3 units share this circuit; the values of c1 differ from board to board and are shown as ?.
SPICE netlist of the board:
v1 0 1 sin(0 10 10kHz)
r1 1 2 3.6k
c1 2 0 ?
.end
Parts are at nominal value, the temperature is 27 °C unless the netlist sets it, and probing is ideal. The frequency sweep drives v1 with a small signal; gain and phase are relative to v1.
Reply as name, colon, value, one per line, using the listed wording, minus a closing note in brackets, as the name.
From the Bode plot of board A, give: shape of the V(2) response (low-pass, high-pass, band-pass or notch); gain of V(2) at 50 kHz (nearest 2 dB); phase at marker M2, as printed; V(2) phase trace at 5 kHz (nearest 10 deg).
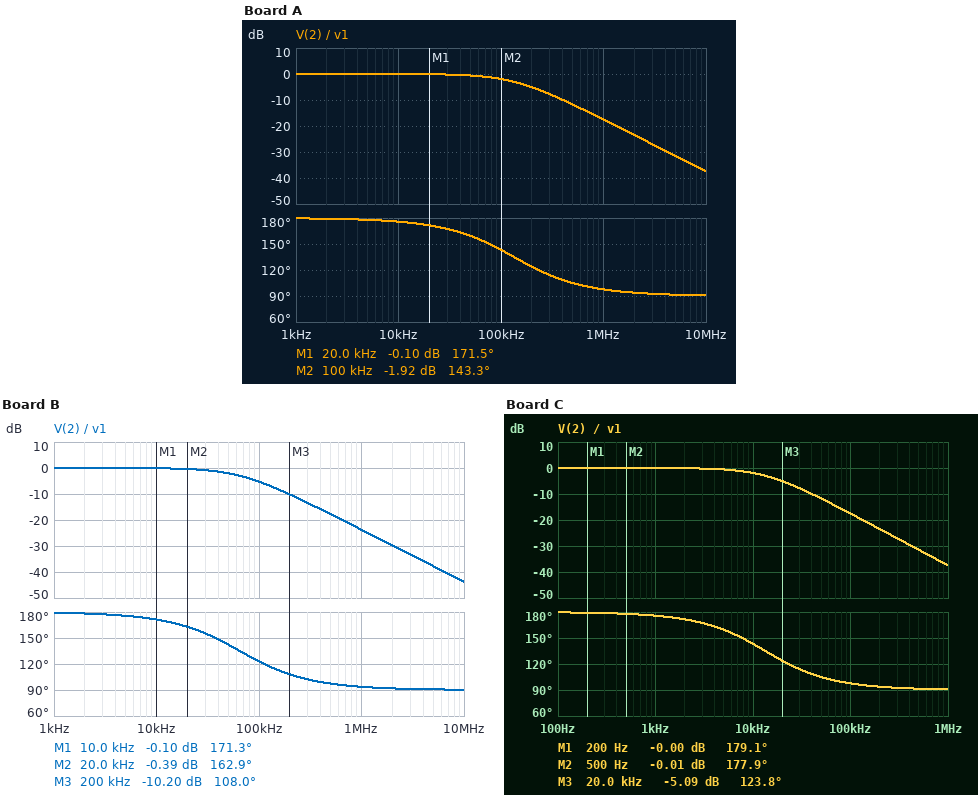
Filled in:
shape of the V(2) response: low-pass
gain of V(2) at 50 kHz: 0 dB
phase at marker M2, as printed: 143.3 deg
V(2) phase trace at 5 kHz: 180 deg
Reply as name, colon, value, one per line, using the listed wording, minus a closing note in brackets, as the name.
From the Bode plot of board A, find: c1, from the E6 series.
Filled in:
c1, from the E6 series: 330 pF
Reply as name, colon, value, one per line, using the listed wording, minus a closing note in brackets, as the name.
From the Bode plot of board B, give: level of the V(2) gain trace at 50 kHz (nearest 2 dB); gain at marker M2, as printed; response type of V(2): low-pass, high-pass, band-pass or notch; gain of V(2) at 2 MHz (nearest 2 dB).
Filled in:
level of the V(2) gain trace at 50 kHz: -2 dB
gain at marker M2, as printed: -0.39 dB
response type of V(2): low-pass, high-pass, band-pass or notch: low-pass
gain of V(2) at 2 MHz: -30 dB
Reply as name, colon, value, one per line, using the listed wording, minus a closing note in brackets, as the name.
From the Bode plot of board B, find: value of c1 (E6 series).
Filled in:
value of c1: 680 pF
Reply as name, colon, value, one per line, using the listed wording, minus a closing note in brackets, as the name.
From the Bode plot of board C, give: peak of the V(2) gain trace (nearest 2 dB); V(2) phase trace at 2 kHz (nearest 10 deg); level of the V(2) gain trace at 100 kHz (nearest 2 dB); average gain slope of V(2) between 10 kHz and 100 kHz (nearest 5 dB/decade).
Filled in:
peak of the V(2) gain trace: 0 dB
V(2) phase trace at 2 kHz: 170 deg
level of the V(2) gain trace at 100 kHz: -18 dB
average gain slope of V(2) between 10 kHz and 100 kHz: -15 dB/decade
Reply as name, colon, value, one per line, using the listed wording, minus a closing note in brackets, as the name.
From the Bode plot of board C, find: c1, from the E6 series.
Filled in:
c1, from the E6 series: 3.3 nF
